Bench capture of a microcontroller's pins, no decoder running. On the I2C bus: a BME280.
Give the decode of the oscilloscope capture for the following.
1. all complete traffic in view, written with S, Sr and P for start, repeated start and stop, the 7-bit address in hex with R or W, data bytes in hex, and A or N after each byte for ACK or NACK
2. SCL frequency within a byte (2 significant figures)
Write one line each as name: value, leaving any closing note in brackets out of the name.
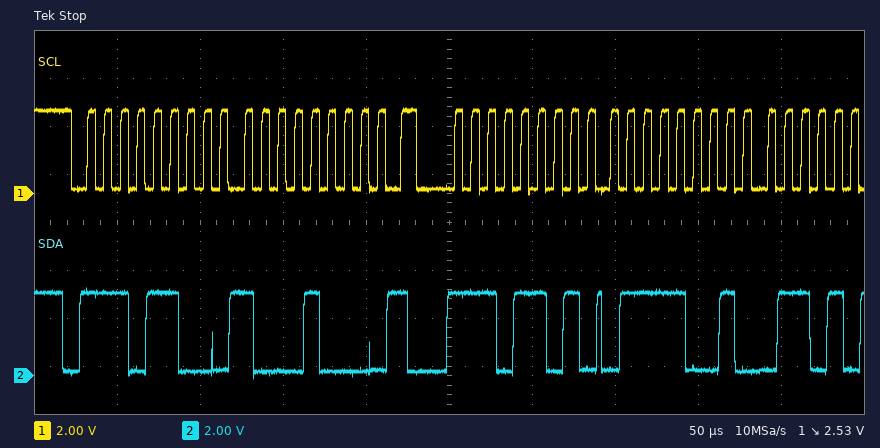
all complete traffic in view, written with S, Sr and P for start, repeated start and stop, the 7-bit address in hex with R or W, data bytes in hex, and A or N after each byte for ACK or NACK: S 76W A 88 A Sr 76R A 79 A
SCL frequency within a byte: 100 kHz
